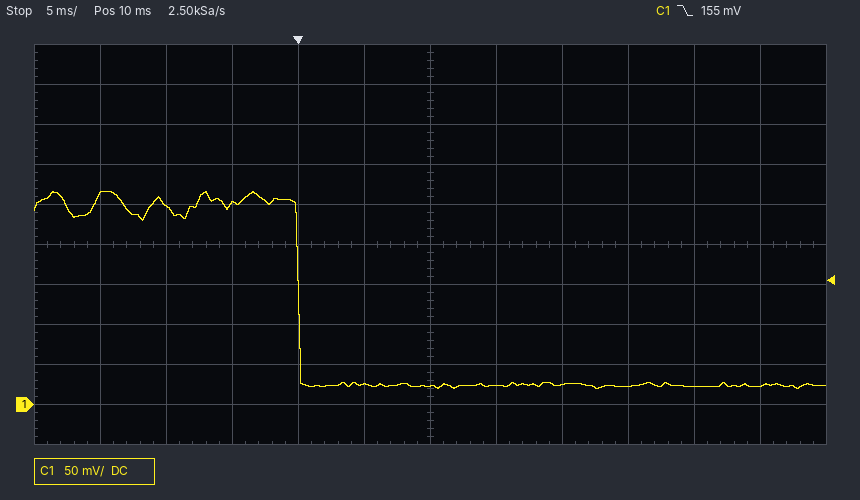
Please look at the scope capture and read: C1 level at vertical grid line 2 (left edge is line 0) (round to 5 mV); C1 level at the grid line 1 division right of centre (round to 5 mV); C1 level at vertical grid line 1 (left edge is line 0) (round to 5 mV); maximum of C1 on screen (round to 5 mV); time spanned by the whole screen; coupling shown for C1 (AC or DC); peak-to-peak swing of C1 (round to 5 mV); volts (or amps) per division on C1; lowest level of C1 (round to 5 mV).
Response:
250 mV
25 mV
260 mV
265 mV
60 ms
DC
245 mV
50 mV
20 mV
